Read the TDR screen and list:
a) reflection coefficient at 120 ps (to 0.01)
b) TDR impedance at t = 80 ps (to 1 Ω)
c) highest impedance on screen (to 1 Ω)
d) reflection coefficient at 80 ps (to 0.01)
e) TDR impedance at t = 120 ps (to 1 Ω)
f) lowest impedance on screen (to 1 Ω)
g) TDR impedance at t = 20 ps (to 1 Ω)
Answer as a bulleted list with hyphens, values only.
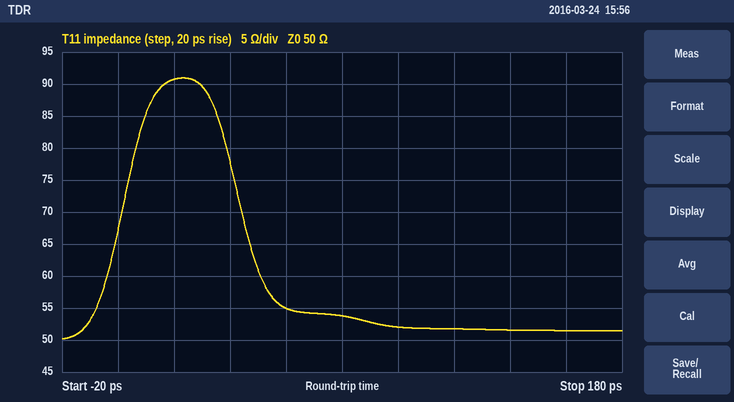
- +0.02
- 54 Ω
- 91 Ω
- +0.04
- 52 Ω
- 50 Ω
- 91 Ω
